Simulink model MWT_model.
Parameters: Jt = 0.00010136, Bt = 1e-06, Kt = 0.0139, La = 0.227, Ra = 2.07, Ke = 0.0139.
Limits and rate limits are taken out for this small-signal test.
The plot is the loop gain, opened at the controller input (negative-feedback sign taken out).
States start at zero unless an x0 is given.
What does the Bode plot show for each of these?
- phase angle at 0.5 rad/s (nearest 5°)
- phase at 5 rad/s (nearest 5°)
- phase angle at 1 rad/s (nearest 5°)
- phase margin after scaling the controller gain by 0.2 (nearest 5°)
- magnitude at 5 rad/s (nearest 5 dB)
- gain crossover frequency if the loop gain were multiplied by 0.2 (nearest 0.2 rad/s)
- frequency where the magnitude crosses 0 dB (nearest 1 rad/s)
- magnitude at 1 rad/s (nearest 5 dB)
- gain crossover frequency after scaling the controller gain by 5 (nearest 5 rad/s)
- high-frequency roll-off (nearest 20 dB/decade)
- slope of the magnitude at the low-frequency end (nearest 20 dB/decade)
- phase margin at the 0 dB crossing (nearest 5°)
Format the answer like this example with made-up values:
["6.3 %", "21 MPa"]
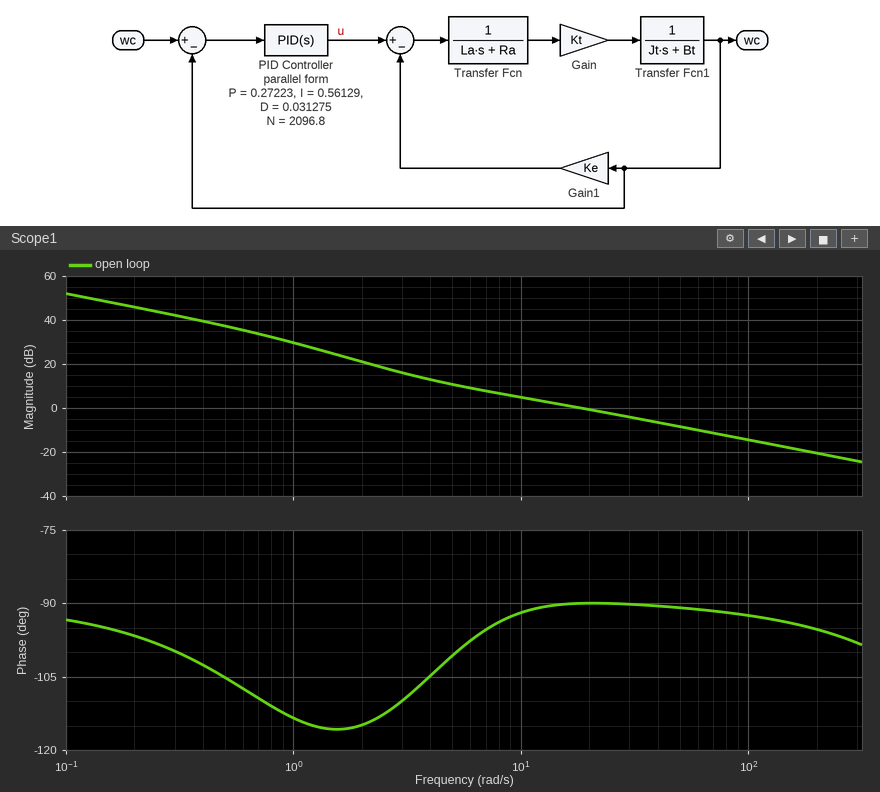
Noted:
["-105°", "-100°", "-115°", "75°", "10 dB", "3.6 rad/s", "18 rad/s", "30 dB", "95 rad/s", "-20 dB/decade", "-20 dB/decade", "90°"]
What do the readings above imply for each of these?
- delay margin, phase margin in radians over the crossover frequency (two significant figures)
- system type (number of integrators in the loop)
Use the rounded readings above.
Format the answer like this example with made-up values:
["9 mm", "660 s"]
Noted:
["0.087 s", "1"]
